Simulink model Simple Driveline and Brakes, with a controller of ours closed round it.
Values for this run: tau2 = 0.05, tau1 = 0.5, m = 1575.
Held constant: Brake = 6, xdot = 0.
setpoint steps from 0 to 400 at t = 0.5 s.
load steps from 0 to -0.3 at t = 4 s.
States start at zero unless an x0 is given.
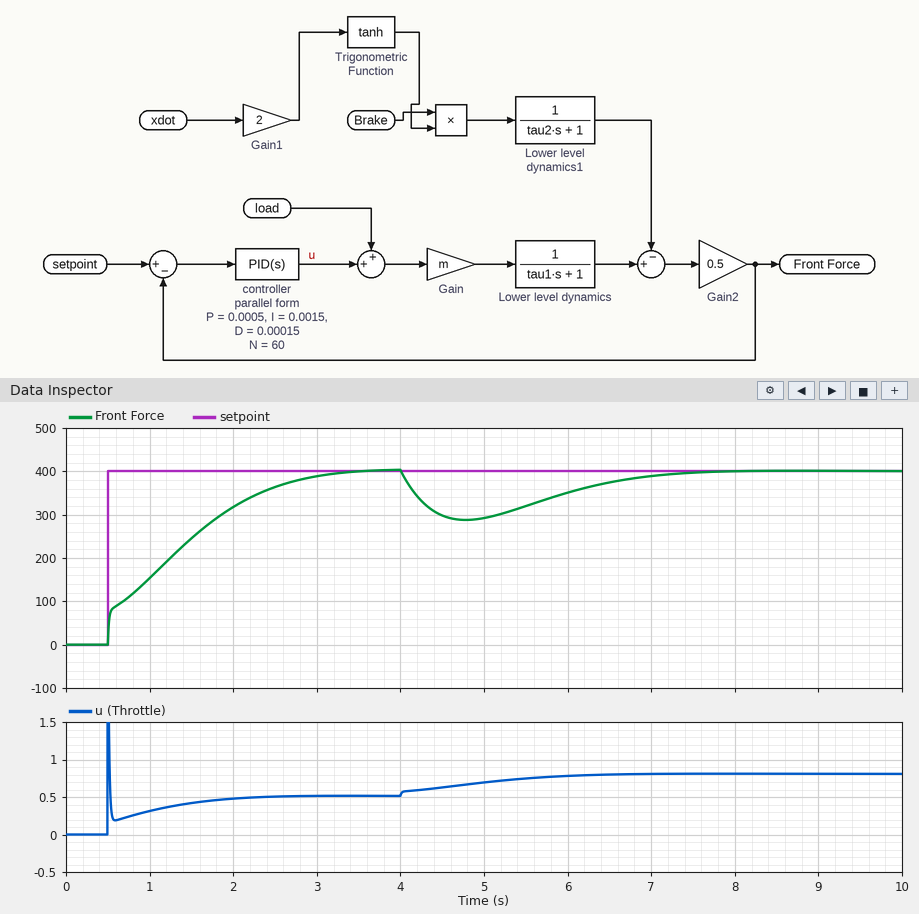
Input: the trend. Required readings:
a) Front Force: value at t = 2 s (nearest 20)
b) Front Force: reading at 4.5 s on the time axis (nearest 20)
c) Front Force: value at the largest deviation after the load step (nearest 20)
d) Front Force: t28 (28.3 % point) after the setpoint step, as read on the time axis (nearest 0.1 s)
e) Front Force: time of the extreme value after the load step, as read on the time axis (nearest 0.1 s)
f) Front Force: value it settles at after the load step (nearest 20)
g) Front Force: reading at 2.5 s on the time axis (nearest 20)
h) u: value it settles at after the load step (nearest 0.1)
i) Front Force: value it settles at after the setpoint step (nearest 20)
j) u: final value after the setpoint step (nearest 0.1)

320
300
280
0.8 s
4.8 s
400
360
0.8
400
0.5
